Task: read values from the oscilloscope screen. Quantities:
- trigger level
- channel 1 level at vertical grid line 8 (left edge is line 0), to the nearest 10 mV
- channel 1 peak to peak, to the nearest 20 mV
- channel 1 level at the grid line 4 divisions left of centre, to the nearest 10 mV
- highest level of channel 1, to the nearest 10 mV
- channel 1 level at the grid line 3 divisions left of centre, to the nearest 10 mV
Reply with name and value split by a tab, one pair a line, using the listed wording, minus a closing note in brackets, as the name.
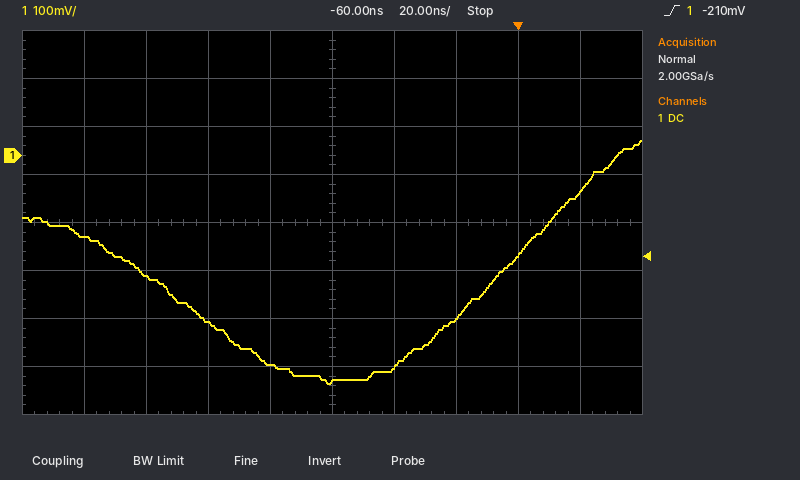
trigger level	-210 mV
channel 1 level at vertical grid line 8 (left edge is line 0), to the nearest 10 mV	-210 mV
channel 1 peak to peak, to the nearest 20 mV	500 mV
channel 1 level at the grid line 4 divisions left of centre, to the nearest 10 mV	-170 mV
highest level of channel 1, to the nearest 10 mV	30 mV
channel 1 level at the grid line 3 divisions left of centre, to the nearest 10 mV	-250 mV
